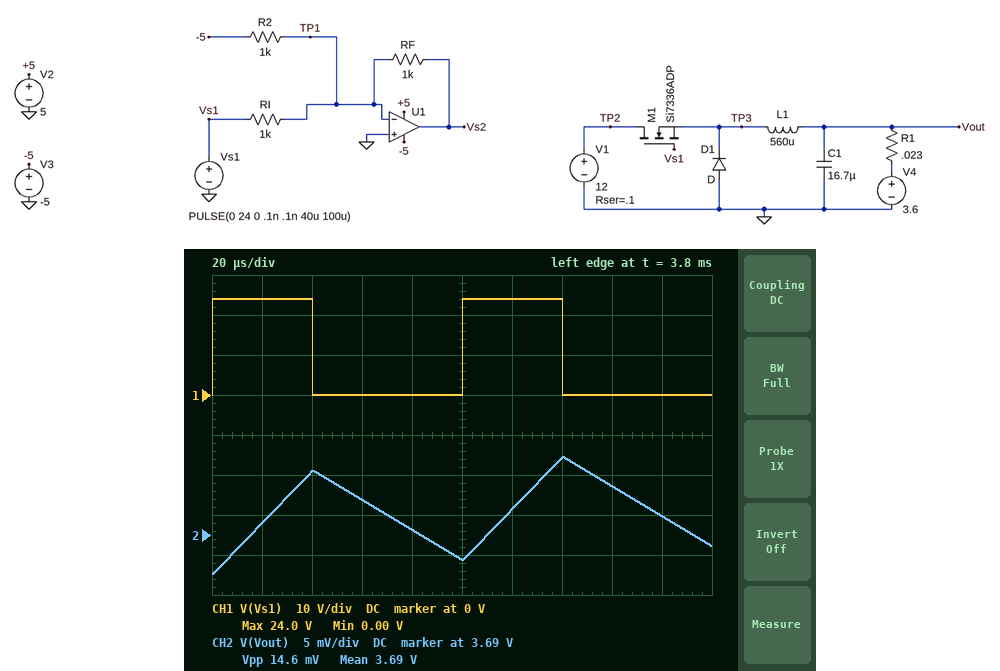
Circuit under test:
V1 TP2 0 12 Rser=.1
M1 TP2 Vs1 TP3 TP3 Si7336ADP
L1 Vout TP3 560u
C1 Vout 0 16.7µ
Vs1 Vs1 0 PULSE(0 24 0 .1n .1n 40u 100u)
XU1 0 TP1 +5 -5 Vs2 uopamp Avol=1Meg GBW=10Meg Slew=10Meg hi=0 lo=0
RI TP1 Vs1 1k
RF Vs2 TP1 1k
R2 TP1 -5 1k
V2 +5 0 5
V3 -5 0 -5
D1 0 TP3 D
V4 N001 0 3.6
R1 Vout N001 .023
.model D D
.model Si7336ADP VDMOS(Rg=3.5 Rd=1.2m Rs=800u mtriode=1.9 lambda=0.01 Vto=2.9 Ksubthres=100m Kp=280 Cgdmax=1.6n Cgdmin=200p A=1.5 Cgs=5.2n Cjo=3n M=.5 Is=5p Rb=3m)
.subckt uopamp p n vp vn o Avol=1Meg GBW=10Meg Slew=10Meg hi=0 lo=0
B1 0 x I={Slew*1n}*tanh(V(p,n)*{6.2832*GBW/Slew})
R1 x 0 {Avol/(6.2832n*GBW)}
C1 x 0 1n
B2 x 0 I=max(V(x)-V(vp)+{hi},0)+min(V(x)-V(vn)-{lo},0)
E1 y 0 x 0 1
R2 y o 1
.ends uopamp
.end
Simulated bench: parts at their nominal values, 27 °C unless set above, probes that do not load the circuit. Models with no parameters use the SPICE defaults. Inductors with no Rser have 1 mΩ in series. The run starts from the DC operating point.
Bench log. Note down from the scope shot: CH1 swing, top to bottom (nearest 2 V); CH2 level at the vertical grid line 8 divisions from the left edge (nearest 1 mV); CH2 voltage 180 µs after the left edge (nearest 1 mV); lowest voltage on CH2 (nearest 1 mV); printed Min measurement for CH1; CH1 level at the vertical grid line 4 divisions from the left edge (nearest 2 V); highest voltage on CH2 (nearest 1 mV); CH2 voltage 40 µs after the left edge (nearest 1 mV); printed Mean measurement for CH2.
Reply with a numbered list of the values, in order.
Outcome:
1. 24 V
2. 3.696 V
3. 3.692 V
4. 3.685 V
5. 0.00 V
6. 0 V
7. 3.700 V
8. 3.698 V
9. 3.69 V
